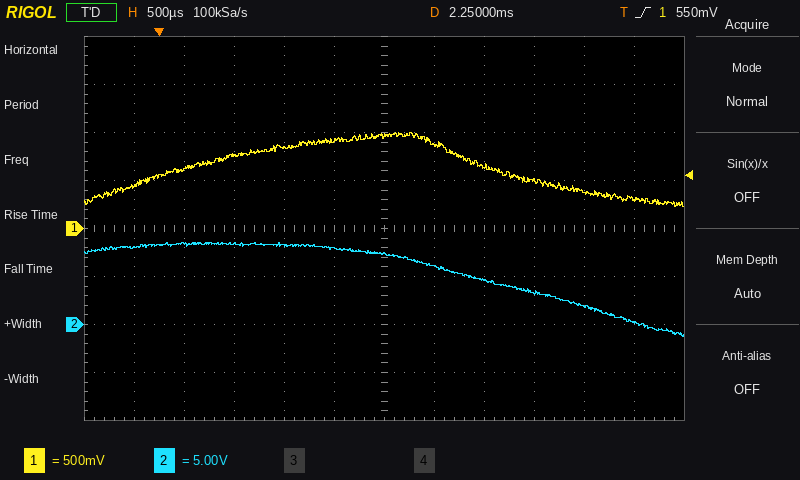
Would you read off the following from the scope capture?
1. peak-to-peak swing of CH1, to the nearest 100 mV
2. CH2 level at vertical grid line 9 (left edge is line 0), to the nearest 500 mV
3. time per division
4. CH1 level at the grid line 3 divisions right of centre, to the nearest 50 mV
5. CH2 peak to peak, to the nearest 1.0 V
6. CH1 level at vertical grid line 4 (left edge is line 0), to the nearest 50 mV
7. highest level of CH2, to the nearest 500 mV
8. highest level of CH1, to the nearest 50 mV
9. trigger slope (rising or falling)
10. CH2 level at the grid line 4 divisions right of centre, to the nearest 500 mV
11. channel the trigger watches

800 mV
3.5 V
500 µs
500 mV
10.0 V
850 mV
8.5 V
1.00 V
rising
2.0 V
CH1
